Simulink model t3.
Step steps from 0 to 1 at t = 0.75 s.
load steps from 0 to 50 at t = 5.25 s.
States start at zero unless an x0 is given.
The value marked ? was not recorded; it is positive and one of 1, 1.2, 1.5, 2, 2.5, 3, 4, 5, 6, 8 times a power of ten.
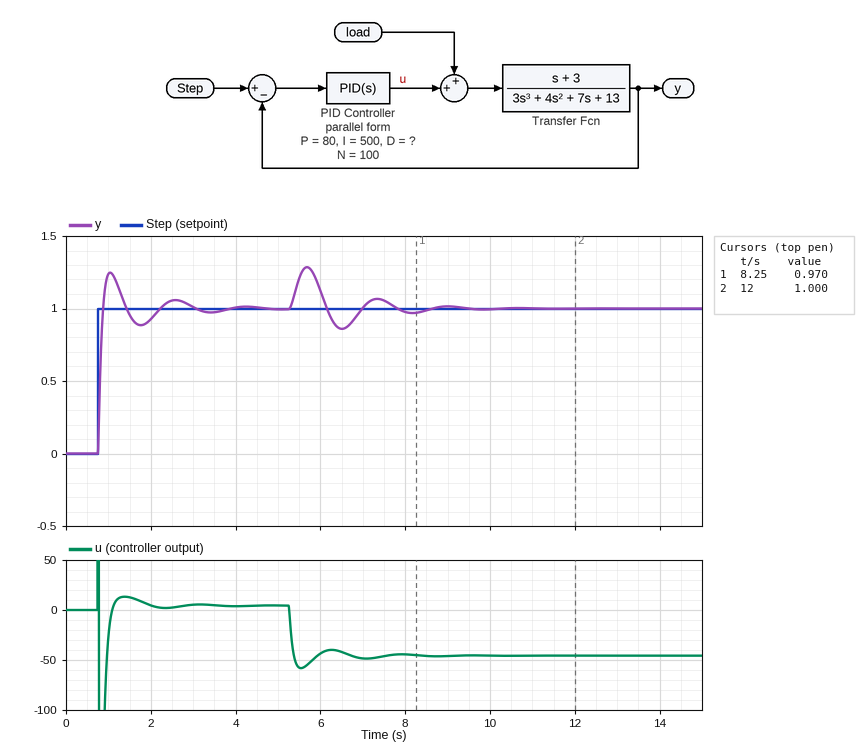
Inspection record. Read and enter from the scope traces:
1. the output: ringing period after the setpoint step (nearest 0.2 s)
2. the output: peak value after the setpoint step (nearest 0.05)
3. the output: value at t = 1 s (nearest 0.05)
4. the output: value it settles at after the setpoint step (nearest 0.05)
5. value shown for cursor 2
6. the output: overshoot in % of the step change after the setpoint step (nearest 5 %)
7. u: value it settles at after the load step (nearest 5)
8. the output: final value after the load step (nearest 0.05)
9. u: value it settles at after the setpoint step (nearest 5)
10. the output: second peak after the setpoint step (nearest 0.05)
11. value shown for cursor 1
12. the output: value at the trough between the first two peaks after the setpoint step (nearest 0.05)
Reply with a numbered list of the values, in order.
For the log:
1. 1.6 s
2. 1.25
3. 1.25
4. 1.00
5. 1.000
6. 25 %
7. -45
8. 1.00
9. 5
10. 1.05
11. 0.970
12. 0.90
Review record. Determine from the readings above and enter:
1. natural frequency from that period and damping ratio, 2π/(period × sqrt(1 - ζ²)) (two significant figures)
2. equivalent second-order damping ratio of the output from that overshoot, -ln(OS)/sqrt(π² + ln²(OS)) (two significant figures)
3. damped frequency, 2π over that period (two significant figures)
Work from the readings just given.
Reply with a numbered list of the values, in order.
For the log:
1. 4.3 rad/s
2. 0.40
3. 3.9 rad/s
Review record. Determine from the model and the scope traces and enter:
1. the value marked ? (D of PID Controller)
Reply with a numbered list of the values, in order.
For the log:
1. 40
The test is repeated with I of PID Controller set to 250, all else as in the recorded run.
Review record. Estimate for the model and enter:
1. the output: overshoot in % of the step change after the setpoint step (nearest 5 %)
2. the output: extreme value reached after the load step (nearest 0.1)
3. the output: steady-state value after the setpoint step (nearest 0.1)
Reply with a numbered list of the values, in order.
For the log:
1. 20 %
2. 1.3
3. 1.0
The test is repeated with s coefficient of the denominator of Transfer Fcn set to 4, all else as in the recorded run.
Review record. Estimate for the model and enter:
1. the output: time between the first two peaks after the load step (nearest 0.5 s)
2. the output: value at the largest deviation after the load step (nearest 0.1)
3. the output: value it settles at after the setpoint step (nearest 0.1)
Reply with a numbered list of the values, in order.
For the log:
1. 1.5 s
2. 1.3
3. 1.0
